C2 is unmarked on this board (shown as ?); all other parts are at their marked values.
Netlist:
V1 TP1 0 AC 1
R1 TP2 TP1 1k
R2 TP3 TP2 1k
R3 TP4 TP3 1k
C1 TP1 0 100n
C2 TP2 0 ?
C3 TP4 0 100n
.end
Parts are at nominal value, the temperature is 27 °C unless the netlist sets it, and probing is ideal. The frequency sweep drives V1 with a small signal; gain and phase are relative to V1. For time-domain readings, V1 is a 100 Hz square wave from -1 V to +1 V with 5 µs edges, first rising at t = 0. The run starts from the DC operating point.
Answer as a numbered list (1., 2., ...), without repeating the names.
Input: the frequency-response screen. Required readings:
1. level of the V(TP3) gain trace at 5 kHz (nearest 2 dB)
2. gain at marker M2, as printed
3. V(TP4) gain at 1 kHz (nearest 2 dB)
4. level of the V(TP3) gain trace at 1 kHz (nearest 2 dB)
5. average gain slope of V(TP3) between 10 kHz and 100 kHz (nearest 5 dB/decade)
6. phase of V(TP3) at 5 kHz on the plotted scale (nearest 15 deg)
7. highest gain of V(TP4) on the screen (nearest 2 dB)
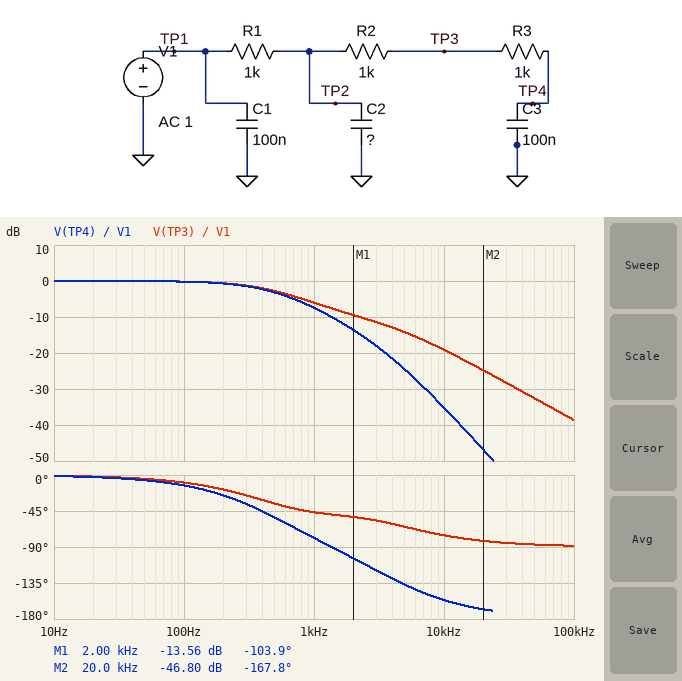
1. -14 dB
2. -46.80 dB
3. -8 dB
4. -6 dB
5. -20 dB/decade
6. -60 deg
7. 0 dB
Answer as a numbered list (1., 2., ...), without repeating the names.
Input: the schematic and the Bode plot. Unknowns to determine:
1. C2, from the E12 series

1. 68 nF
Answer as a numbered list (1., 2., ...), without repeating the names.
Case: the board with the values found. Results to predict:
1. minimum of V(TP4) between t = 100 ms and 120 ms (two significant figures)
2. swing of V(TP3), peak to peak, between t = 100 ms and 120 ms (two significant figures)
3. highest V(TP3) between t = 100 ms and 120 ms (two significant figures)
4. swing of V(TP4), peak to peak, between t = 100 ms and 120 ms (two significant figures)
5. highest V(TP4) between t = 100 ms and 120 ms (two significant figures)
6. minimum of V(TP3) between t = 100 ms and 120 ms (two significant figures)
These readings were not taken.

1. -1.0 V
2. 2.0 V
3. 1.0 V
4. 2.0 V
5. 1.0 V
6. -1.0 V
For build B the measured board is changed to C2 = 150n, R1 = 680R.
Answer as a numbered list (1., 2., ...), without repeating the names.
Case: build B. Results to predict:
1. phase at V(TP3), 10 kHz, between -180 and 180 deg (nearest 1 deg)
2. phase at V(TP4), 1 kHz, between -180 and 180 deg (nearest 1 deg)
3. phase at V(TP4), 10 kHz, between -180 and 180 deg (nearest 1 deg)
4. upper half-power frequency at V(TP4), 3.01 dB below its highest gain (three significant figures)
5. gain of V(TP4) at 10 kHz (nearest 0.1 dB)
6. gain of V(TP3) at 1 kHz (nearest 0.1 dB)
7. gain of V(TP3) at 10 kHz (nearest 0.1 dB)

1. -83 deg
2. -85 deg
3. -164 deg
4. 503 Hz
5. -38.4 dB
6. -5.9 dB
7. -22.3 dB
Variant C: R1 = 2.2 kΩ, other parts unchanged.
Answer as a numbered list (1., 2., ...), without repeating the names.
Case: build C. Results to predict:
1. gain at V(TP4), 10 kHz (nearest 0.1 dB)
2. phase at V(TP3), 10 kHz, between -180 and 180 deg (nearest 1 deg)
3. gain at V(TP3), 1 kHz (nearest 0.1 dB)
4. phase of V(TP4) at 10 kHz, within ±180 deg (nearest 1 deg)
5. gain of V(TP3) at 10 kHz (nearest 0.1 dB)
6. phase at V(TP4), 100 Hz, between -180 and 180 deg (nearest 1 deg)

1. -41.8 dB
2. -82 deg
3. -9.6 dB
4. -163 deg
5. -25.7 dB
6. -20 deg
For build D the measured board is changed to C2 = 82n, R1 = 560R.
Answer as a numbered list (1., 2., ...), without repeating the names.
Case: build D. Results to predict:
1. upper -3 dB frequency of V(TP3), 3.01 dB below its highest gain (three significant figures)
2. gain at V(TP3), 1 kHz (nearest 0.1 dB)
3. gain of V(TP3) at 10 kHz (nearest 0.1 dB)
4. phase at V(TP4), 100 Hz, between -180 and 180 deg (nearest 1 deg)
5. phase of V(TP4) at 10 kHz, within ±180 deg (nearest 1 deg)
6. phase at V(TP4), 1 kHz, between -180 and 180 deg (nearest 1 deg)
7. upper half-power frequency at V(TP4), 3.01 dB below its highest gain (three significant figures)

1. 683 Hz
2. -4.6 dB
3. -16.0 dB
4. -11 deg
5. -152 deg
6. -71 deg
7. 585 Hz
